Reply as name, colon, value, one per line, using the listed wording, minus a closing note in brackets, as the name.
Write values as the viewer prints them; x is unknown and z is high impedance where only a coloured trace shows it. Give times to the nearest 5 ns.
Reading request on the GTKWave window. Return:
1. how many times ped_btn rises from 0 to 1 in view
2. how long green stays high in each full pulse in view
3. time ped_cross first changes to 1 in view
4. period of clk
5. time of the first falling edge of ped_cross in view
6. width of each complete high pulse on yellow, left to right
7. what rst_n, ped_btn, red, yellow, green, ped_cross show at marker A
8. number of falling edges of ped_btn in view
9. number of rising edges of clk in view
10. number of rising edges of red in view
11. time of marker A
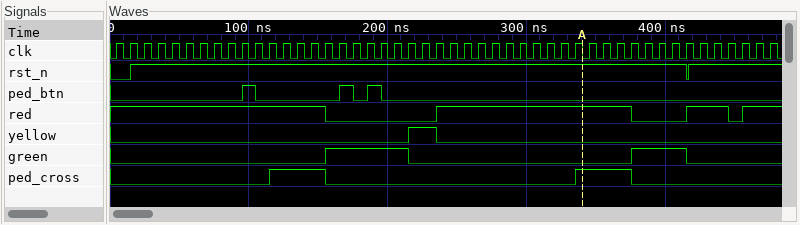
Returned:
how many times ped_btn rises from 0 to 1 in view: 3
how long green stays high in each full pulse in view: 60 ns, 40 ns
time ped_cross first changes to 1 in view: 115 ns
period of clk: 10 ns
time of the first falling edge of ped_cross in view: 155 ns
width of each complete high pulse on yellow, left to right: 20 ns
what rst_n, ped_btn, red, yellow, green, ped_cross show at marker A: rst_n=1, ped_btn=0, red=1, yellow=0, green=0, ped_cross=1
number of falling edges of ped_btn in view: 3
number of rising edges of clk in view: 48
number of rising edges of red in view: 3
time of marker A: 340 ns
